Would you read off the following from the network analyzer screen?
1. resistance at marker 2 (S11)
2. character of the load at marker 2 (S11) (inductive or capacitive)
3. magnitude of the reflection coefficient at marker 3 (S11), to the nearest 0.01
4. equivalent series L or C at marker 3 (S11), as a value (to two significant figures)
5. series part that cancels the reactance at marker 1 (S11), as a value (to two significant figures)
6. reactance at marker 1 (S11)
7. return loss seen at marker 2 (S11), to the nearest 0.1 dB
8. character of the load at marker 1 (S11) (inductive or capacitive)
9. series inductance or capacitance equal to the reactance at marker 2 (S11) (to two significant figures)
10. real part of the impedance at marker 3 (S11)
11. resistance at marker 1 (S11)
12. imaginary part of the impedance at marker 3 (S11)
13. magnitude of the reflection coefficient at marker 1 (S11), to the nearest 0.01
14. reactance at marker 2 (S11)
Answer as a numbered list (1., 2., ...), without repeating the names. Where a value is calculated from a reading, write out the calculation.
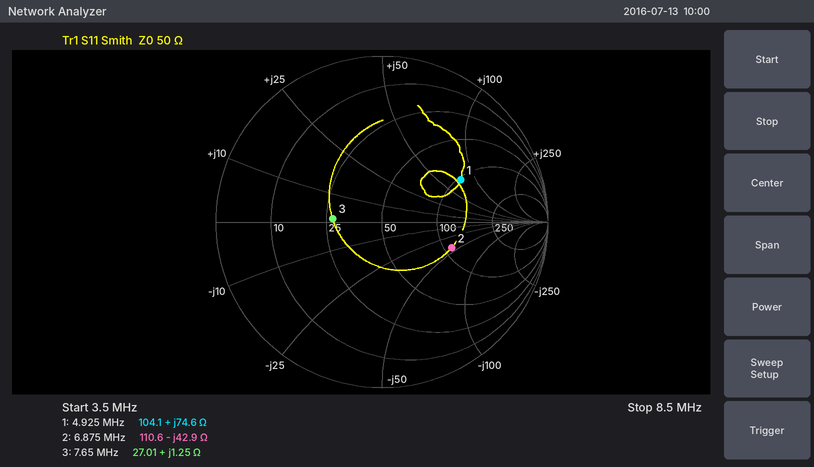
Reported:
1. 110.6 Ω
2. capacitive
3. 0.30
4. L = 1.25 Ω/(2π × 7.65 MHz) ≈ 26 nH
5. C = 1/(2π × 4.925 MHz × 74.6 Ω) ≈ 433 pF, so 430 pF to two significant figures
6. +74.6 Ω
7. 7.0 dB
8. inductive
9. C = 1/(2π × 6.875 MHz × 42.9 Ω) ≈ 540 pF
10. 27.01 Ω
11. 104.1 Ω
12. +1.25 Ω
13. 0.54
14. -42.9 Ω
